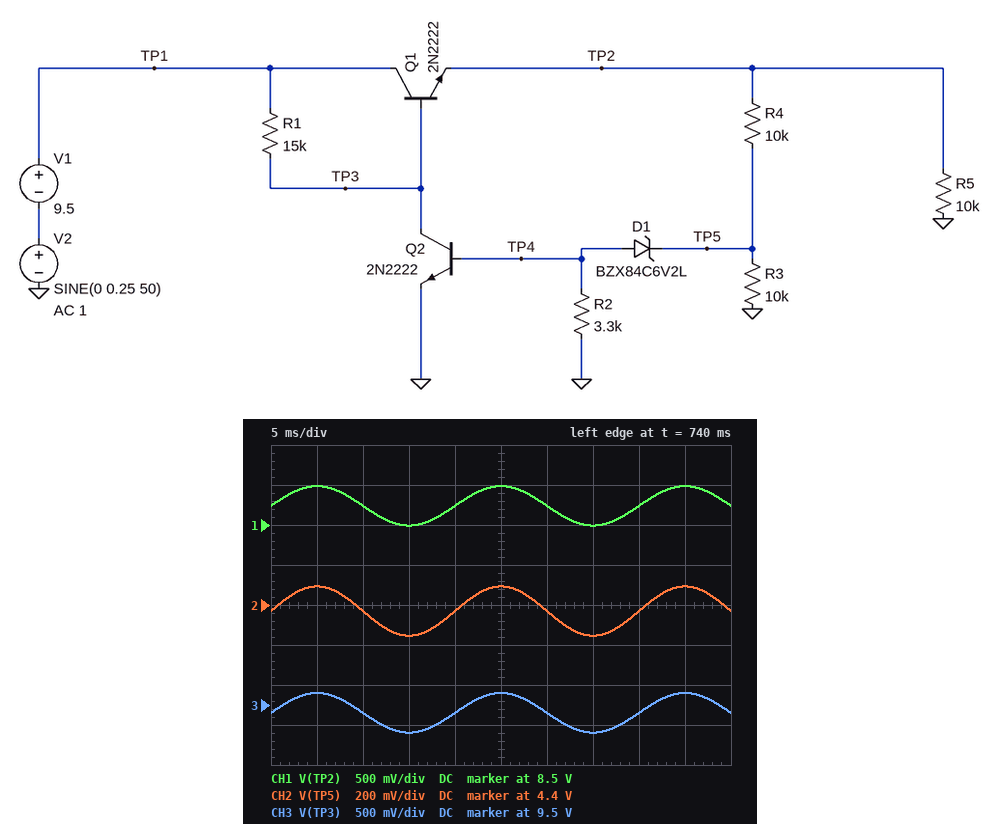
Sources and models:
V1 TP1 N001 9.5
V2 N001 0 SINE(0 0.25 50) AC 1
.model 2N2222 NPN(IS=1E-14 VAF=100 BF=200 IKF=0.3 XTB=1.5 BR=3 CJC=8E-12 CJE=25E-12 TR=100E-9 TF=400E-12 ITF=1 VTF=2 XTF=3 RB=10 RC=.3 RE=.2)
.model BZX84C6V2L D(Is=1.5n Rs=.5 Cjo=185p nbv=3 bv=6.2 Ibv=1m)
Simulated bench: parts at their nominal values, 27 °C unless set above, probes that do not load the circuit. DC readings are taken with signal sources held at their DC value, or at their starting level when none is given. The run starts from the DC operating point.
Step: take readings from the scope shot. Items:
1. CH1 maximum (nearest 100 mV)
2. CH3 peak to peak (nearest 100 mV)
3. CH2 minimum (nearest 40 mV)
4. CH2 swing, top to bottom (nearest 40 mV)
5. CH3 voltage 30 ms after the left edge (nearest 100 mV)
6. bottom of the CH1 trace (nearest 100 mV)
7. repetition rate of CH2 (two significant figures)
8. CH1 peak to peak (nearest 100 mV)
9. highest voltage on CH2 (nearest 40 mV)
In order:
9.0 V
500 mV
4.24 V
240 mV
9.4 V
8.5 V
50 Hz
500 mV
4.48 V
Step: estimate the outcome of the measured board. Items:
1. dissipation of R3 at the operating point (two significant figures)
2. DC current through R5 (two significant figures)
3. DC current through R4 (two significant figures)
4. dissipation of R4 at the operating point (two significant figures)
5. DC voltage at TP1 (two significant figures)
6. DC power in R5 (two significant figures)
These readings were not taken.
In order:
1.9 mW
870 µA
440 µA
1.9 mW
9.5 V
7.6 mW
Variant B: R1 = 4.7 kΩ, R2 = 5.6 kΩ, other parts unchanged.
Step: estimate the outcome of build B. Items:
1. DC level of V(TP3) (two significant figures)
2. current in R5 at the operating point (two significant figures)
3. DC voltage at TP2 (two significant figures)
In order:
9.5 V
880 µA
8.8 V
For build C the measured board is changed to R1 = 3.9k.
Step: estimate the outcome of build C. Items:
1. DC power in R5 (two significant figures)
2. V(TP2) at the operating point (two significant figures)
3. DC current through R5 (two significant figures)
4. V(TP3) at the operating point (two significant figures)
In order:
7.8 mW
8.8 V
880 µA
9.5 V
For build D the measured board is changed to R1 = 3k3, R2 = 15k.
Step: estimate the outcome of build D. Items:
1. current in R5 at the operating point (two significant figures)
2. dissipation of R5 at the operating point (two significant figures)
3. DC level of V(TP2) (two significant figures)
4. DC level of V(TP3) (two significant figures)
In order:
880 µA
7.8 mW
8.8 V
9.5 V
